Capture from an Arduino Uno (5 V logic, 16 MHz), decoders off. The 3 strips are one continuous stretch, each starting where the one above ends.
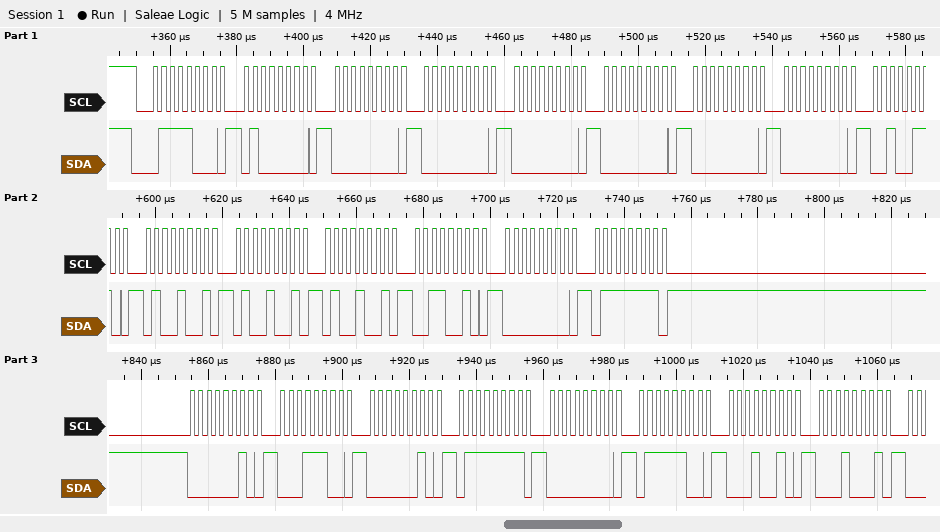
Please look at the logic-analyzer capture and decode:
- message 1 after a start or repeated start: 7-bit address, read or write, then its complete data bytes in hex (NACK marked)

0x3C write: 40 00 00 00 00 00 00 26 49 49 49 32 00 7F 02 1C 02 7F 00 7C 12 11
